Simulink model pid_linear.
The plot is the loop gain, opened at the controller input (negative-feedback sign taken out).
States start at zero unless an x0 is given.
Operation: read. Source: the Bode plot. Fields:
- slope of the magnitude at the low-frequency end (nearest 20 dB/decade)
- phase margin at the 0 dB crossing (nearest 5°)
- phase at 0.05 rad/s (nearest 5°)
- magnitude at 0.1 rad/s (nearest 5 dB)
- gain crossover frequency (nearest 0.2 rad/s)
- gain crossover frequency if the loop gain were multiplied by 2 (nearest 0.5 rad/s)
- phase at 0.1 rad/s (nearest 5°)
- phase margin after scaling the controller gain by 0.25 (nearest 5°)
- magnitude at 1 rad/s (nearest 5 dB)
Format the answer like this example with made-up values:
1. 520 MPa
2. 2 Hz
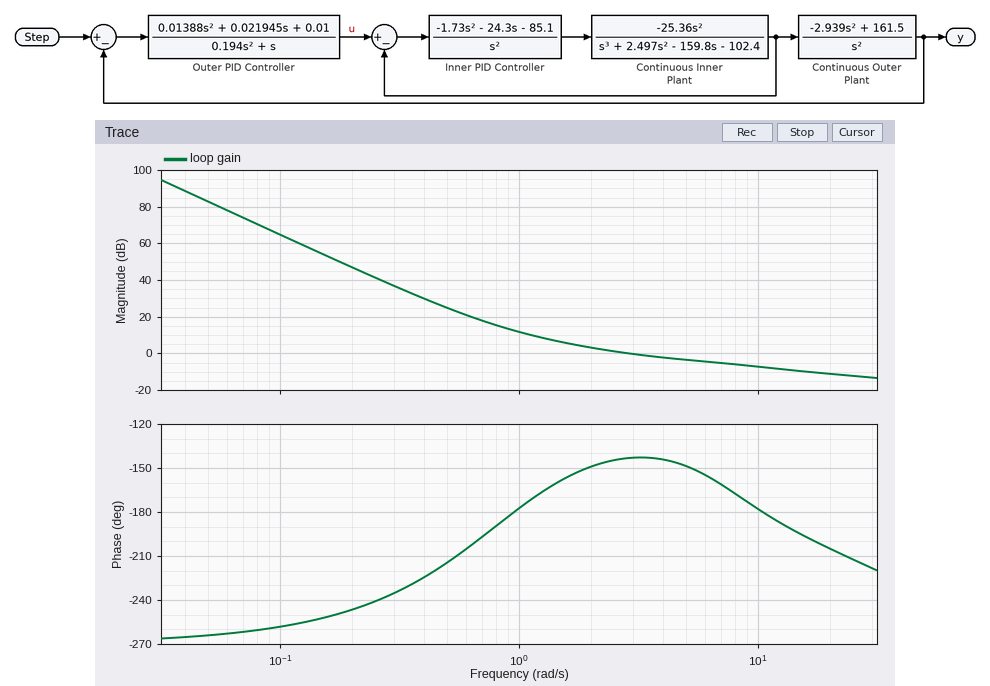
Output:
1. -60 dB/decade
2. 35°
3. -265°
4. 65 dB
5. 2.8 rad/s
6. 8.0 rad/s
7. -260°
8. 0°
9. 10 dB
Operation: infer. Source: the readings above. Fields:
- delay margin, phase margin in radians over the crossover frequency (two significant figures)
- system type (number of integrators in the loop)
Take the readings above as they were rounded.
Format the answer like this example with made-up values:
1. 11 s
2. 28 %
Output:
1. 0.22 s
2. 3
